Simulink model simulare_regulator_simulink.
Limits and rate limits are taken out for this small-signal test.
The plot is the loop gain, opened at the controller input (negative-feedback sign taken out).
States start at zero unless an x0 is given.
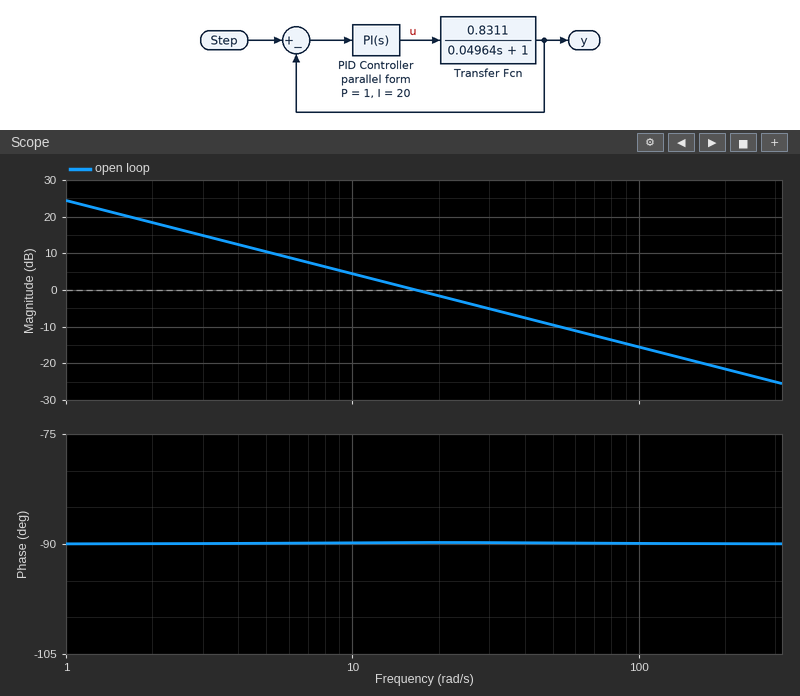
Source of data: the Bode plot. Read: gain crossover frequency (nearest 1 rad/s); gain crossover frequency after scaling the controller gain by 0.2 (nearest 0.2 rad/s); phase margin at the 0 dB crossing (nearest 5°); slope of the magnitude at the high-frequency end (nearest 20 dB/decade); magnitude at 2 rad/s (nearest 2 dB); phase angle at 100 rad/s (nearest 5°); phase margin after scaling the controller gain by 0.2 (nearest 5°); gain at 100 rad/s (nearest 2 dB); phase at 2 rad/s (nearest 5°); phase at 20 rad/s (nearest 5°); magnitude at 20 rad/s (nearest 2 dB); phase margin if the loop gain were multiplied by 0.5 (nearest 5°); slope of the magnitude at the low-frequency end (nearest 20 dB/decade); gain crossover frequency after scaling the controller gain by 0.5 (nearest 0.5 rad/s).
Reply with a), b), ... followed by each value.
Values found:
a) 17 rad/s
b) 3.4 rad/s
c) 90°
d) -20 dB/decade
e) 18 dB
f) -90°
g) 90°
h) -16 dB
i) -90°
j) -90°
k) -2 dB
l) 90°
m) -20 dB/decade
n) 8.5 rad/s
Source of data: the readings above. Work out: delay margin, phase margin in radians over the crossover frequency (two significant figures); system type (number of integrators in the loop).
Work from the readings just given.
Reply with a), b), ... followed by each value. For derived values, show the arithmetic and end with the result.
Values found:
a) 90 × π / 180 / 17 = 0.092 s
b) 1
